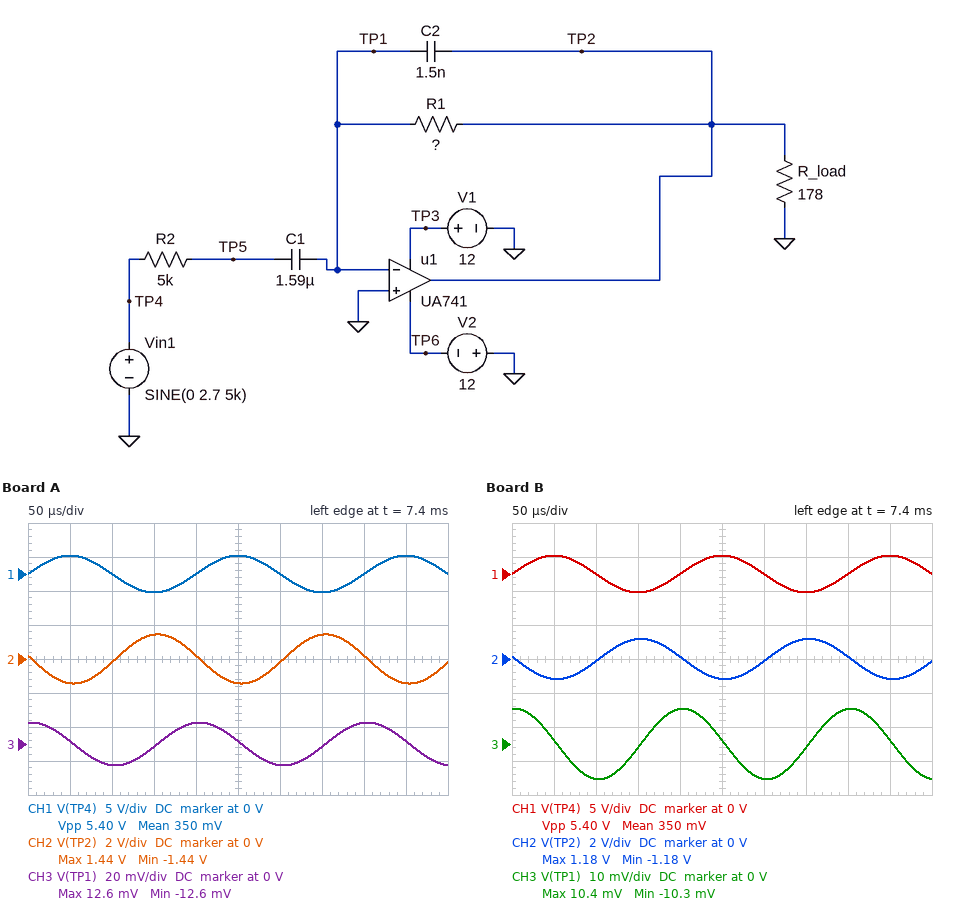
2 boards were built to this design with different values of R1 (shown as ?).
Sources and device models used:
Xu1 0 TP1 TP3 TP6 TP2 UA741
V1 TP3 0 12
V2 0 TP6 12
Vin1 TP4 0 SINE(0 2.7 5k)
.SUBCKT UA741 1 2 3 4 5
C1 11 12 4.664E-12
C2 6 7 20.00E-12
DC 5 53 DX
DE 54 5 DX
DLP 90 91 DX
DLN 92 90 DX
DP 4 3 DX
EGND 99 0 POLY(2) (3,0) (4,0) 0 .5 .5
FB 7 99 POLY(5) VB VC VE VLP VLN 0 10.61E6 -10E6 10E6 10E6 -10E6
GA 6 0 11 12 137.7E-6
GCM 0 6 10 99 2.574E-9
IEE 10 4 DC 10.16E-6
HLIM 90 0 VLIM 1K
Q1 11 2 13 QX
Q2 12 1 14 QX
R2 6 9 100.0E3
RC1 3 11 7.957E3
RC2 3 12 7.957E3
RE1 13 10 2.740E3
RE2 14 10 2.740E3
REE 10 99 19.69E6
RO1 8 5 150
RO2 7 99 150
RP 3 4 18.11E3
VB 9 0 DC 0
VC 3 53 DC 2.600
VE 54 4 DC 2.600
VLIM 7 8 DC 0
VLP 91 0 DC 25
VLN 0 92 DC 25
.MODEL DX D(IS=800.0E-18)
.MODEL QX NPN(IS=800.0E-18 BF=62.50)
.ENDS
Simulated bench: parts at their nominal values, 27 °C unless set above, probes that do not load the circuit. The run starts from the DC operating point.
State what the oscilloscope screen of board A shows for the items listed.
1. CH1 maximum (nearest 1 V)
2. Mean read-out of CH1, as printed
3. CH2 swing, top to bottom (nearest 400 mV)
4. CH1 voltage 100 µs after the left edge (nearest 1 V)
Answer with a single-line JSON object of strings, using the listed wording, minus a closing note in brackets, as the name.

{"CH1 maximum": "3 V", "Mean read-out of CH1, as printed": "350 mV", "CH2 swing, top to bottom": "2.8 V", "CH1 voltage 100 µs after the left edge": "0 V"}
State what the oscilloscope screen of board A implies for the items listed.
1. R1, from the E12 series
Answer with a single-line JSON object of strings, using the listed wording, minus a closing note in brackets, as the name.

{"R1, from the E12 series": "2.7 kΩ"}
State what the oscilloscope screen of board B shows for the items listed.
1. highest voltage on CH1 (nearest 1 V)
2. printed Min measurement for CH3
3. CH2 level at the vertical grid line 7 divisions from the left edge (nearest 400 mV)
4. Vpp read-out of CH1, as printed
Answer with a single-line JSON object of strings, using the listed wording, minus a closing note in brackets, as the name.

{"highest voltage on CH1": "3 V", "printed Min measurement for CH3": "-10.3 mV", "CH2 level at the vertical grid line 7 divisions from the left edge": "1.2 V", "Vpp read-out of CH1, as printed": "5.40 V"}
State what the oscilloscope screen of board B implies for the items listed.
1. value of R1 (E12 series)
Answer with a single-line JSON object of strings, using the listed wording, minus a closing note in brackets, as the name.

{"value of R1": "2.2 kΩ"}
